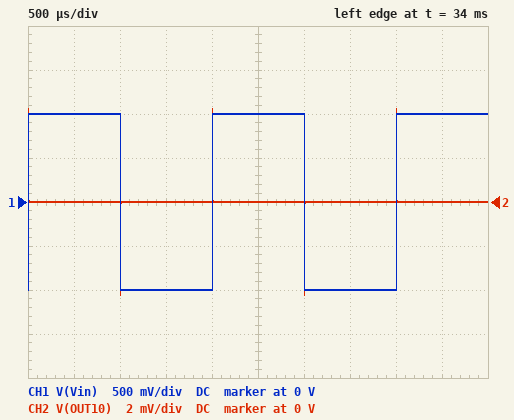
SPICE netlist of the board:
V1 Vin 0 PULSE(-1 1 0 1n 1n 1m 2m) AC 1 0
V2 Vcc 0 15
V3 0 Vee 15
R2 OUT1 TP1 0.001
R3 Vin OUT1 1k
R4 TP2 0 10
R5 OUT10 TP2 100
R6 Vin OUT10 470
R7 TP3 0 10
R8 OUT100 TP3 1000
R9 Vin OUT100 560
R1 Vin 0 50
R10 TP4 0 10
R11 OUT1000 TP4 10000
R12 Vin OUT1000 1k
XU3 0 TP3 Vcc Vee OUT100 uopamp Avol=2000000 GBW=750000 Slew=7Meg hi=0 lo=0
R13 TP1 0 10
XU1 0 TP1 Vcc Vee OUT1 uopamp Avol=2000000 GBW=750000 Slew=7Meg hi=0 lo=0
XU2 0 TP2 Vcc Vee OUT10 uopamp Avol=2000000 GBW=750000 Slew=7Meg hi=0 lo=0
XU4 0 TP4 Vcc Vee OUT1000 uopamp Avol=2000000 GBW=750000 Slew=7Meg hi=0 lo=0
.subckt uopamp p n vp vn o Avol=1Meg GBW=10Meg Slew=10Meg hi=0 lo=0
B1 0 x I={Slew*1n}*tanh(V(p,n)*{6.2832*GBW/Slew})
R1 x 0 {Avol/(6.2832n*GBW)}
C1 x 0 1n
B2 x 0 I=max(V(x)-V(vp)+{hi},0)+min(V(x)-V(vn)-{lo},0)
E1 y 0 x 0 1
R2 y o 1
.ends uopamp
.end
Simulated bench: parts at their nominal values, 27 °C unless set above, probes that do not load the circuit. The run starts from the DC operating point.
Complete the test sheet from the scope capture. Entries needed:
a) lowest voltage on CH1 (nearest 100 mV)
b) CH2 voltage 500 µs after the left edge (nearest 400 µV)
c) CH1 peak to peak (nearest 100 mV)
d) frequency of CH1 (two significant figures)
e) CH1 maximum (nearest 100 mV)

-1.0 V
0 V
2.0 V
500 Hz
1.0 V
